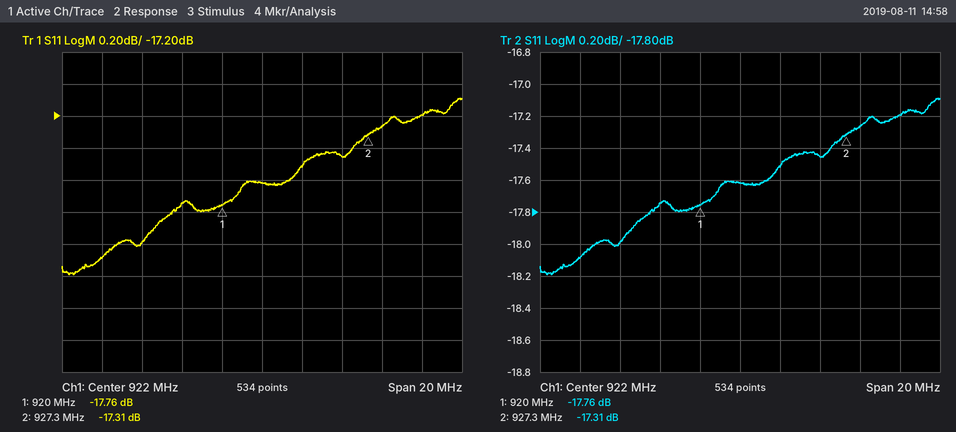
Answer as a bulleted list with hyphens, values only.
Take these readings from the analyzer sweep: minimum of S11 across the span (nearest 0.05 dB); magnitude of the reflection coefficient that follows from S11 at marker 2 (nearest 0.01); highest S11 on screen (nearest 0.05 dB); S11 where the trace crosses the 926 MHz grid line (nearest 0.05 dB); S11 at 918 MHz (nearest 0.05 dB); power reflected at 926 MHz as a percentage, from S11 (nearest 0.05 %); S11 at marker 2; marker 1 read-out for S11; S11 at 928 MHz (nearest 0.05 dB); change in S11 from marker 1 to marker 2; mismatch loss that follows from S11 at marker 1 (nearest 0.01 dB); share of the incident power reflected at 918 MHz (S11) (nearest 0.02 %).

- -18.20 dB
- 0.14
- -17.10 dB
- -17.45 dB
- -17.75 dB
- 1.80 %
- -17.31 dB
- -17.76 dB
- -17.25 dB
- 0.45 dB
- 0.07 dB
- 1.68 %
